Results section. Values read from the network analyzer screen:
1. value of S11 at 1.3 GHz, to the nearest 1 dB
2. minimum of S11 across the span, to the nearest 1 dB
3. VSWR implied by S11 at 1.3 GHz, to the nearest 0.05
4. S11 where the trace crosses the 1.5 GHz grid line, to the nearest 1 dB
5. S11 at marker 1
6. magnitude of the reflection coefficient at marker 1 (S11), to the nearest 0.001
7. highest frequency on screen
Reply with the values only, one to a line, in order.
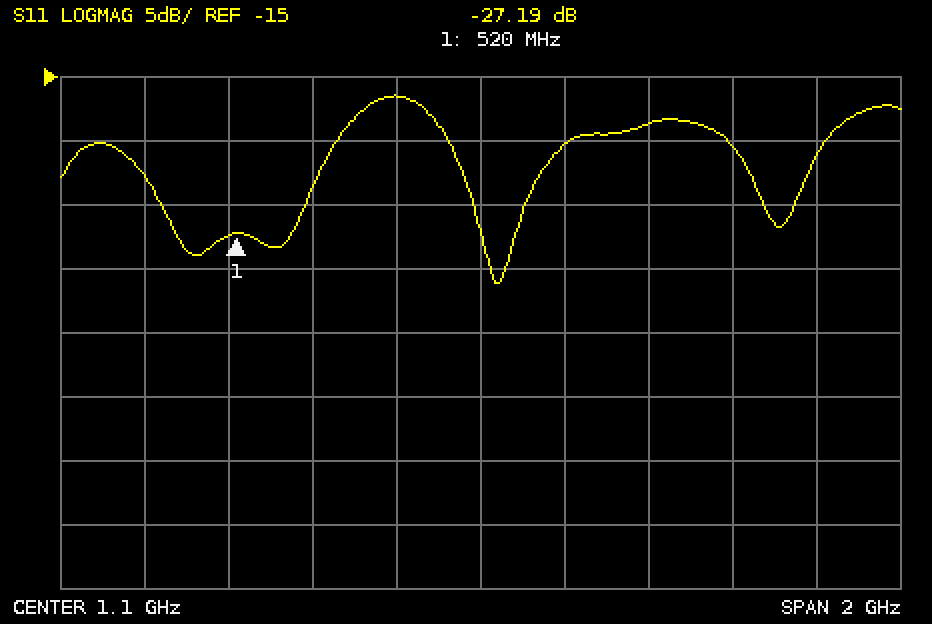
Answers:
-20 dB
-31 dB
1.20
-19 dB
-27.19 dB
0.044
2.1 GHz
